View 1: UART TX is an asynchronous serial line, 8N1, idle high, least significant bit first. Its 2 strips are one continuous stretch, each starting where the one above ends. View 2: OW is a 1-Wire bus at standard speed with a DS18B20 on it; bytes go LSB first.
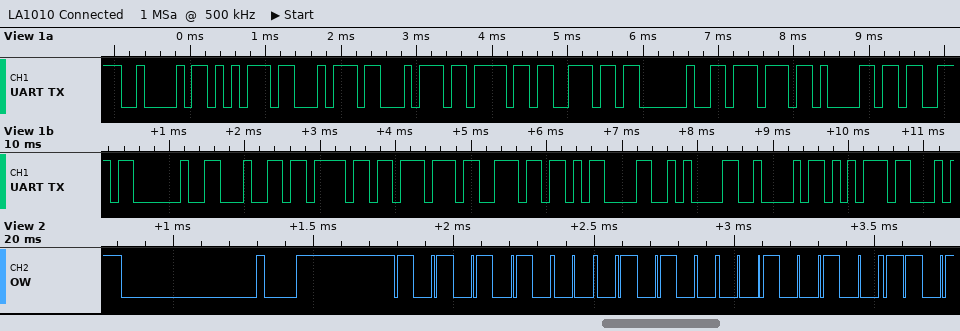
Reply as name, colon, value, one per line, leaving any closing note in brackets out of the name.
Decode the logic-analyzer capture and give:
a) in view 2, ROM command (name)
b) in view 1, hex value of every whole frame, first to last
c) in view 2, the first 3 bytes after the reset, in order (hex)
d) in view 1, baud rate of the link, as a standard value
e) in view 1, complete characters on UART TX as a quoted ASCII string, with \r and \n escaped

in view 2, ROM command: Match ROM
in view 1, hex value of every whole frame, first to last: 0x42 0x75 0x74 0x74 0x6F 0x6E 0x20 0x77 0x61 0x73 0x20 0x64 0x6F 0x77 0x6E 0x0D 0x0A 0x42 0x75
in view 2, the first 3 bytes after the reset, in order: 55 28 24
in view 1, baud rate of the link, as a standard value: 9600 baud
in view 1, complete characters on UART TX as a quoted ASCII string, with \r and \n escaped: "Button was down\r\nBu"
